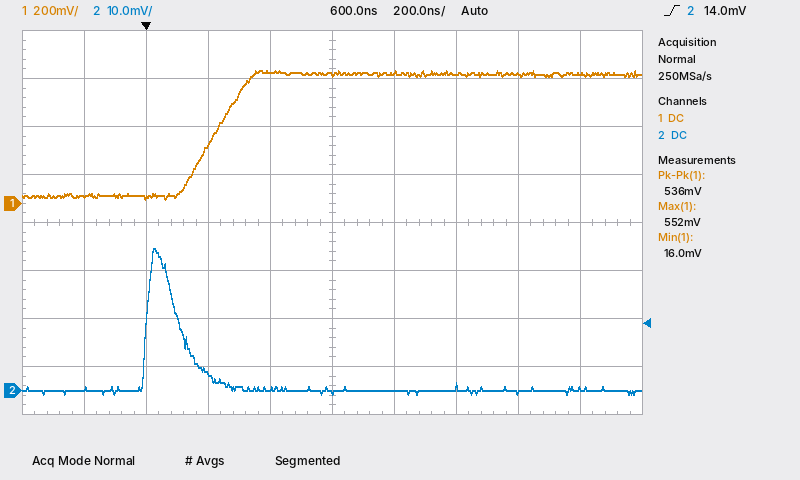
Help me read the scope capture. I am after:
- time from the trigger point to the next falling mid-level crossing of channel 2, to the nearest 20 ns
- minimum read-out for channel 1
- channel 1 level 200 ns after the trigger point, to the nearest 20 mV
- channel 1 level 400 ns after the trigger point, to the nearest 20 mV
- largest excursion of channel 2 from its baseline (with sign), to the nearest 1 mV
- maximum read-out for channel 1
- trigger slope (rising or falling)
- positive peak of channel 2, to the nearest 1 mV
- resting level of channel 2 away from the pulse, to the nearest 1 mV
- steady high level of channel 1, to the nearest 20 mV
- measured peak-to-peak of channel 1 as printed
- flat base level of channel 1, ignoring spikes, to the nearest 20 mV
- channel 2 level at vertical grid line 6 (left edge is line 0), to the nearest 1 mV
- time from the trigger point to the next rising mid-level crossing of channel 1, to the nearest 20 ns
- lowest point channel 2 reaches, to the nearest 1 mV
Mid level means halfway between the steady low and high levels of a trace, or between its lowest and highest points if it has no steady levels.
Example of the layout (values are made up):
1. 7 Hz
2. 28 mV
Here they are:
1. 100 ns
2. 16.0 mV
3. 240 mV
4. 540 mV
5. +30 mV
6. 552 mV
7. rising
8. 30 mV
9. 0 mV
10. 540 mV
11. 536 mV
12. 40 mV
13. 0 mV
14. 220 ns
15. -1 mV
